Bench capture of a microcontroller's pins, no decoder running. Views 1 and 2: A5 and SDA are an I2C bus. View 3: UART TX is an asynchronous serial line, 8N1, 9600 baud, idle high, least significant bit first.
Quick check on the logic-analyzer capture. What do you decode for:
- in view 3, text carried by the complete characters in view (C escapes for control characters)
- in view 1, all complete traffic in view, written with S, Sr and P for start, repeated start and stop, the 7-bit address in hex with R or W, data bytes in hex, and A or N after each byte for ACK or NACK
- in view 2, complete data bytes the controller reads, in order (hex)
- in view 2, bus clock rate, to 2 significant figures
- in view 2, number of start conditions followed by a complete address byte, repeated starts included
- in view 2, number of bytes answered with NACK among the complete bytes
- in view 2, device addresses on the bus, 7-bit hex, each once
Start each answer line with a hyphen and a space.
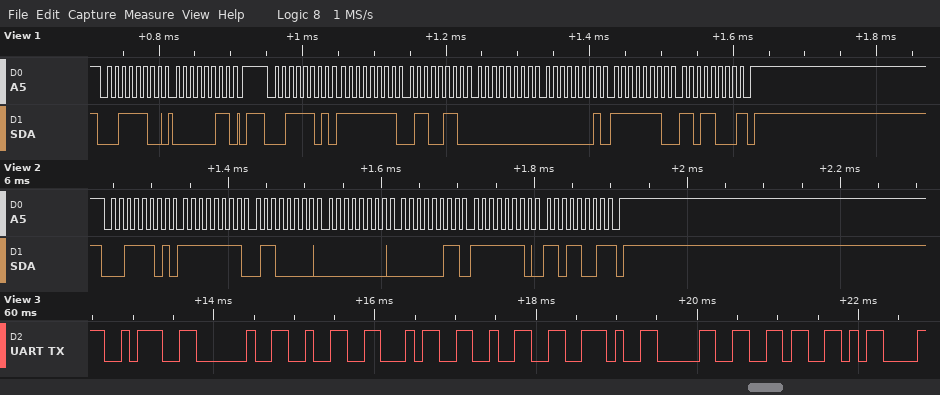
- ": 242.06\r"
- S 1EW A 03 A P S 1ER A FF A 66 A 00 A 01 A FE A D8 N P
- FF 60 00 03 FE D9
- 100 kHz
- 1
- 1
- 0x1E
